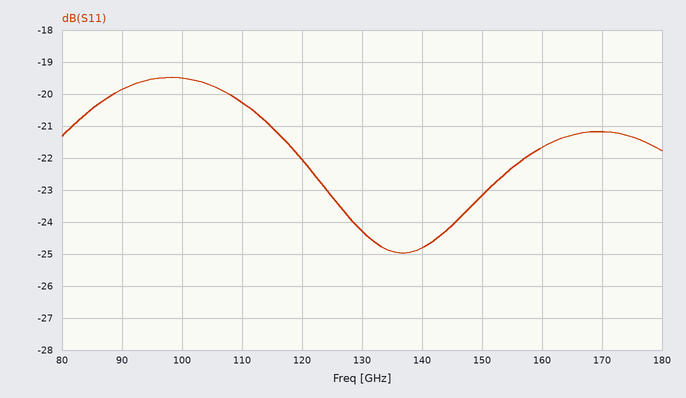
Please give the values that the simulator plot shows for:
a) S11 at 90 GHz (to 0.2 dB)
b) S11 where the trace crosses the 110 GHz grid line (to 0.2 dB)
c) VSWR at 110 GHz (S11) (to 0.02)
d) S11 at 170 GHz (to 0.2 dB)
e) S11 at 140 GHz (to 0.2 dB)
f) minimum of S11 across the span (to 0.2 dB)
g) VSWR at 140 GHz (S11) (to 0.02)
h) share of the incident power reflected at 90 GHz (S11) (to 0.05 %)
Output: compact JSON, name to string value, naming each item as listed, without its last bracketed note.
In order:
{"S11 at 90 GHz": "-19.8 dB", "S11 where the trace crosses the 110 GHz grid line": "-20.2 dB", "VSWR at 110 GHz (S11)": "1.22", "S11 at 170 GHz": "-21.2 dB", "S11 at 140 GHz": "-24.8 dB", "minimum of S11 across the span": "-25.0 dB", "VSWR at 140 GHz (S11)": "1.12", "share of the incident power reflected at 90 GHz (S11)": "1.05 %"}
